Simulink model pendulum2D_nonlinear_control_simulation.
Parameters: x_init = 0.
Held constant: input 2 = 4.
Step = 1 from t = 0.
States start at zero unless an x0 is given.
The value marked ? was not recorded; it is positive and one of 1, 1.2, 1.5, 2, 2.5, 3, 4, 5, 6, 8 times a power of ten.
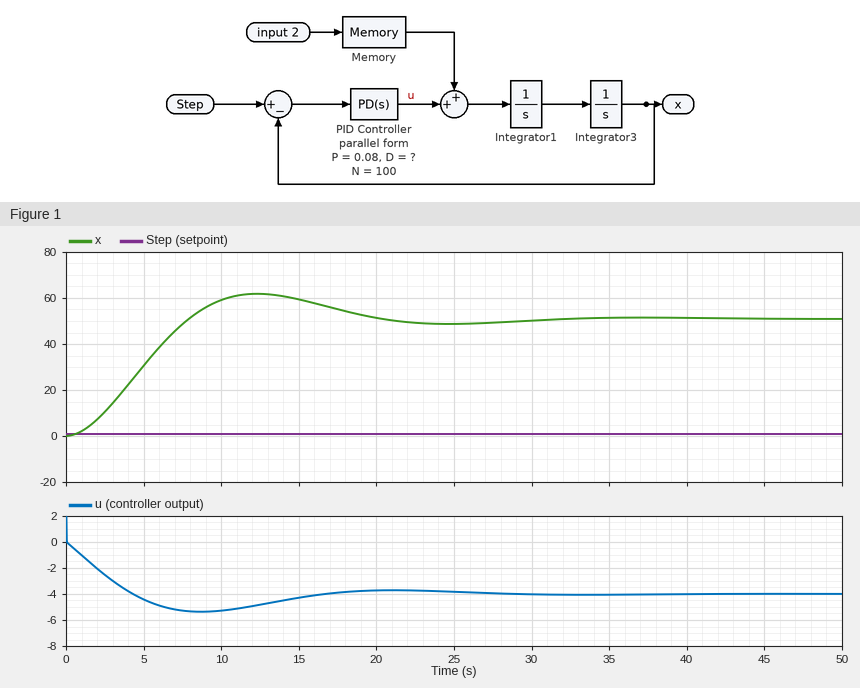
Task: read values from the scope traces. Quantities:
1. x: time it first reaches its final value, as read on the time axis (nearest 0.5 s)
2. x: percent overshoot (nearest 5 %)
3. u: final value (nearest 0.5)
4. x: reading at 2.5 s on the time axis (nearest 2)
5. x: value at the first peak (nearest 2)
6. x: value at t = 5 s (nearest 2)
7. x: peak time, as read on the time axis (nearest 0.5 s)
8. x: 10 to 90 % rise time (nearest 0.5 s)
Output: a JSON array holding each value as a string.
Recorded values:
["8.0 s", "20 %", "-4.0", "10", "62", "30", "12.5 s", "5.5 s"]
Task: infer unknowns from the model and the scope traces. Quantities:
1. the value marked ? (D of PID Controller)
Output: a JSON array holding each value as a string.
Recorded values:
["0.25"]
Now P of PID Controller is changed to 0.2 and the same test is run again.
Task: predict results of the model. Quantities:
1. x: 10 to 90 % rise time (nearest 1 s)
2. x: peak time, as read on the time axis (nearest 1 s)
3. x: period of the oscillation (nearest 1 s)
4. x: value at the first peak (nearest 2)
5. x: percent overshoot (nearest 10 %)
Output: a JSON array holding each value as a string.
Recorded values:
["3 s", "7 s", "15 s", "30", "40 %"]
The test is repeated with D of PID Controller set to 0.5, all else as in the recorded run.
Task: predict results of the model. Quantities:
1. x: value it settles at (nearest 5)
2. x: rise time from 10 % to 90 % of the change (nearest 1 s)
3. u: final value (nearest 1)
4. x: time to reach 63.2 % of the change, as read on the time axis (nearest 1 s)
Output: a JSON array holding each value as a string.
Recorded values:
["50", "10 s", "-4", "7 s"]
